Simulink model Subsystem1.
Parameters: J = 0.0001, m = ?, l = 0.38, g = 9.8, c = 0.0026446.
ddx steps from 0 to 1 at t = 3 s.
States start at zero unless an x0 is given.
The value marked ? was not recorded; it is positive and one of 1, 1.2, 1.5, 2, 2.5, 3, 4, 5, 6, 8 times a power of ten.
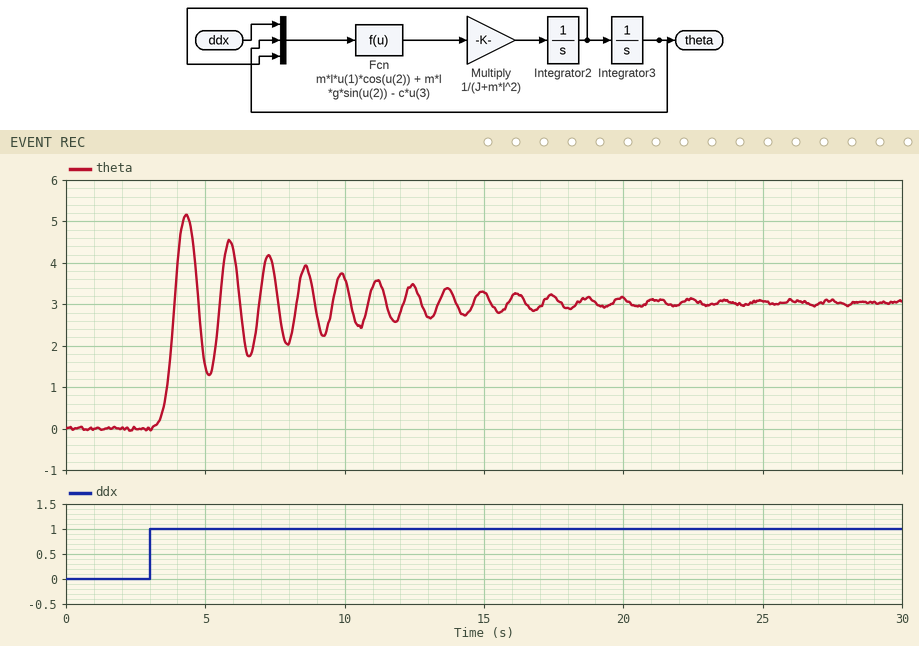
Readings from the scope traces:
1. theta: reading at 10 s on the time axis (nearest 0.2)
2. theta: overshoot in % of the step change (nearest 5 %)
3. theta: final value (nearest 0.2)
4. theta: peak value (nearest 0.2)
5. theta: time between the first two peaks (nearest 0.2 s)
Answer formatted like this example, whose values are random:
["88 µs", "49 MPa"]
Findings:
["3.6", "70 %", "3.0", "5.2", "1.6 s"]
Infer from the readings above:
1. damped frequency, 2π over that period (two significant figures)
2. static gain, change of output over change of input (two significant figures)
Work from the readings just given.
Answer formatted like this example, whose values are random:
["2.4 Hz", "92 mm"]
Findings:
["3.9 rad/s", "3.0"]
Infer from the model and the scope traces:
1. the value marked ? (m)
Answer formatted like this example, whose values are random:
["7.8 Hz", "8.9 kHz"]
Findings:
["0.05"]
